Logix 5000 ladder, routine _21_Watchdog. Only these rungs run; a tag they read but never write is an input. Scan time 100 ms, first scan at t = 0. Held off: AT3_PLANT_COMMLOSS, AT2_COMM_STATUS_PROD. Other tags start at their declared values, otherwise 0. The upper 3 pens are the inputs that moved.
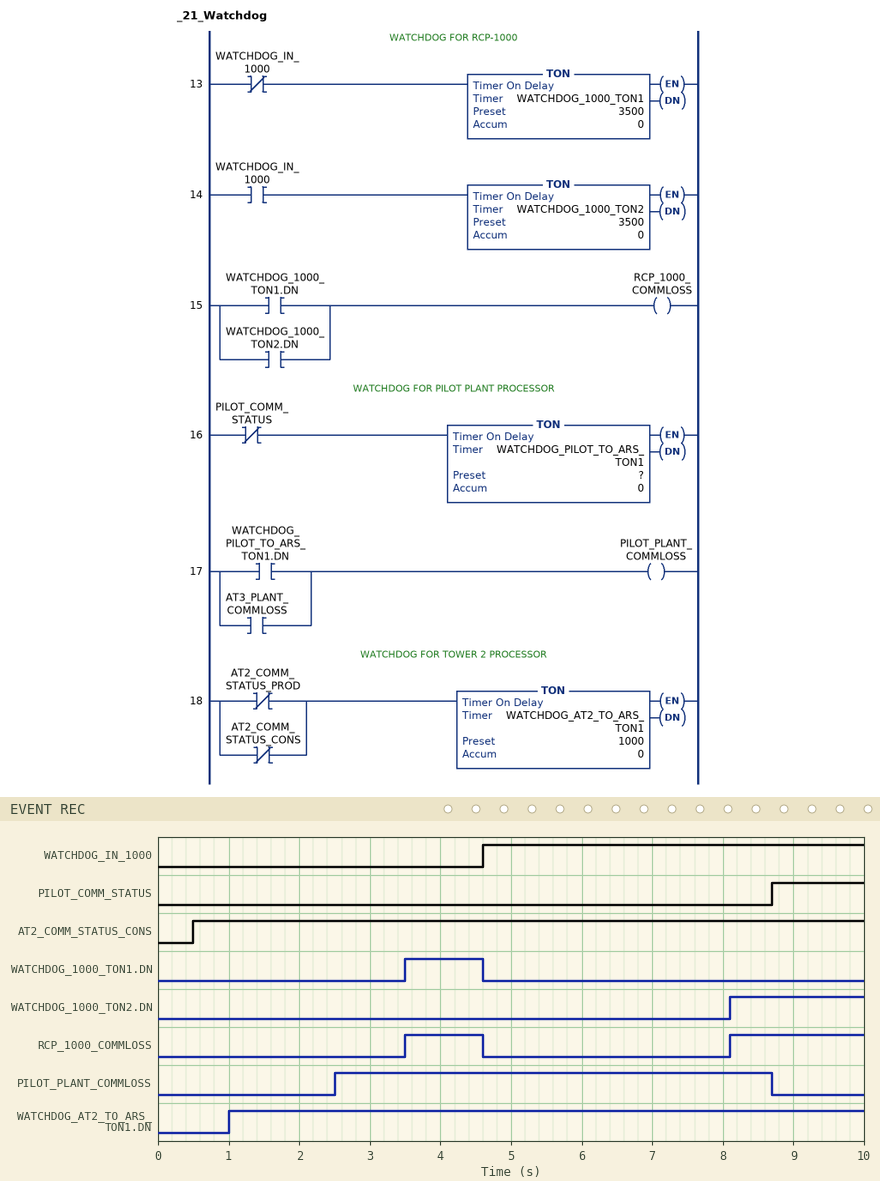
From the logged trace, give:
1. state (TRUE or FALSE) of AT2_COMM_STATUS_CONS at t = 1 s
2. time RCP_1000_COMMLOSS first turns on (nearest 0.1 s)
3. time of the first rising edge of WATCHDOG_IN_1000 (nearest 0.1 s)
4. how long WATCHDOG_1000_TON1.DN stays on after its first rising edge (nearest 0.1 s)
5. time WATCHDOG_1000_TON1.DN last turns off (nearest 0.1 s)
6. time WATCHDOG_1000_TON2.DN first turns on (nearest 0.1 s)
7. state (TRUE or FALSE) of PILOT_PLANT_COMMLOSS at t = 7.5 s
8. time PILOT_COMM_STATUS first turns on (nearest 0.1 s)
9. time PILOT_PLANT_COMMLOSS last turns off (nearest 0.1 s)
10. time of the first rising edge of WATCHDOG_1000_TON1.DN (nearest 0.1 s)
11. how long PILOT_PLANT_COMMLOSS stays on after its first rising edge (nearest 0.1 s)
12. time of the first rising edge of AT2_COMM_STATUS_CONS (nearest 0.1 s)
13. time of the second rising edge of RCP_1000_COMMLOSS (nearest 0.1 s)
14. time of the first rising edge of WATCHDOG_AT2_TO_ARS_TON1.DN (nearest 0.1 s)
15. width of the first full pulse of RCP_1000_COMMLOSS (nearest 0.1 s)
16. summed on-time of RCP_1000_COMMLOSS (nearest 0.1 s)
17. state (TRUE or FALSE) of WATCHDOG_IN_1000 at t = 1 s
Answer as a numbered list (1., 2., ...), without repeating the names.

1. TRUE
2. 3.5 s
3. 4.6 s
4. 1.1 s
5. 4.6 s
6. 8.1 s
7. TRUE
8. 8.7 s
9. 8.7 s
10. 3.5 s
11. 6.2 s
12. 0.5 s
13. 8.1 s
14. 1.0 s
15. 1.1 s
16. 3.0 s
17. FALSE
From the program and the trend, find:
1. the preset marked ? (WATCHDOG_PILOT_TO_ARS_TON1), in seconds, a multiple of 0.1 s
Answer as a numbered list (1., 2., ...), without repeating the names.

1. 2.5 s
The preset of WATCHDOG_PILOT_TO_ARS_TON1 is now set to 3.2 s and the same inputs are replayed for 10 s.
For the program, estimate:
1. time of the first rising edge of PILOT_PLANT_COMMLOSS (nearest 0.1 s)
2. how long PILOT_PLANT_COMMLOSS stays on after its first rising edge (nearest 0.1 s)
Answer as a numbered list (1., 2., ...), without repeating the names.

1. 3.2 s
2. 5.5 s
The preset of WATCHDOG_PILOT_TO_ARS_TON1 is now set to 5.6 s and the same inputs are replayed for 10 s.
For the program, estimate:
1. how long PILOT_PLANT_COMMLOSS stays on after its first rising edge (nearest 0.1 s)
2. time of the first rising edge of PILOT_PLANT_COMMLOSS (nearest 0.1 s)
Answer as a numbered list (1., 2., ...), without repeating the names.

1. 3.1 s
2. 5.6 s
